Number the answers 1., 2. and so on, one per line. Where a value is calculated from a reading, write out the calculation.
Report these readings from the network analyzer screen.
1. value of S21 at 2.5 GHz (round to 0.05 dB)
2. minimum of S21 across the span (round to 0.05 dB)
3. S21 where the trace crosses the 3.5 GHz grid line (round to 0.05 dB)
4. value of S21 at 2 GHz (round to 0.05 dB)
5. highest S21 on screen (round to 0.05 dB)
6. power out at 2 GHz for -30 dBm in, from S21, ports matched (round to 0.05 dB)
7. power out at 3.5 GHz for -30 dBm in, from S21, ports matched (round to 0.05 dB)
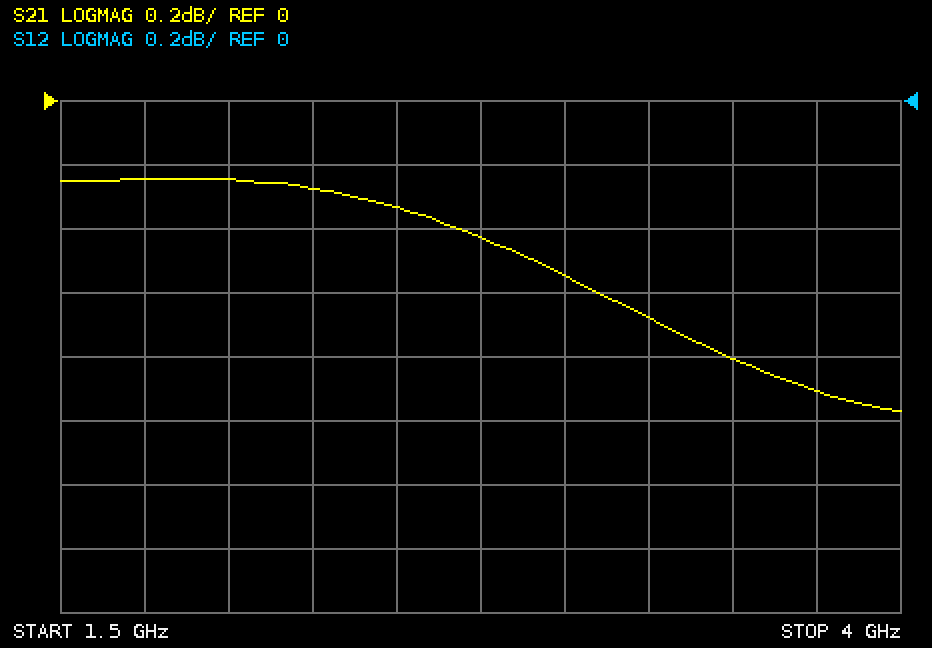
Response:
1. -0.35 dB
2. -0.95 dB
3. -0.80 dB
4. -0.25 dB
5. -0.25 dB
6. -30 dBm + (-0.25 dB) = -30.25 dBm
7. -30 dBm + (-0.80 dB) = -30.80 dBm
